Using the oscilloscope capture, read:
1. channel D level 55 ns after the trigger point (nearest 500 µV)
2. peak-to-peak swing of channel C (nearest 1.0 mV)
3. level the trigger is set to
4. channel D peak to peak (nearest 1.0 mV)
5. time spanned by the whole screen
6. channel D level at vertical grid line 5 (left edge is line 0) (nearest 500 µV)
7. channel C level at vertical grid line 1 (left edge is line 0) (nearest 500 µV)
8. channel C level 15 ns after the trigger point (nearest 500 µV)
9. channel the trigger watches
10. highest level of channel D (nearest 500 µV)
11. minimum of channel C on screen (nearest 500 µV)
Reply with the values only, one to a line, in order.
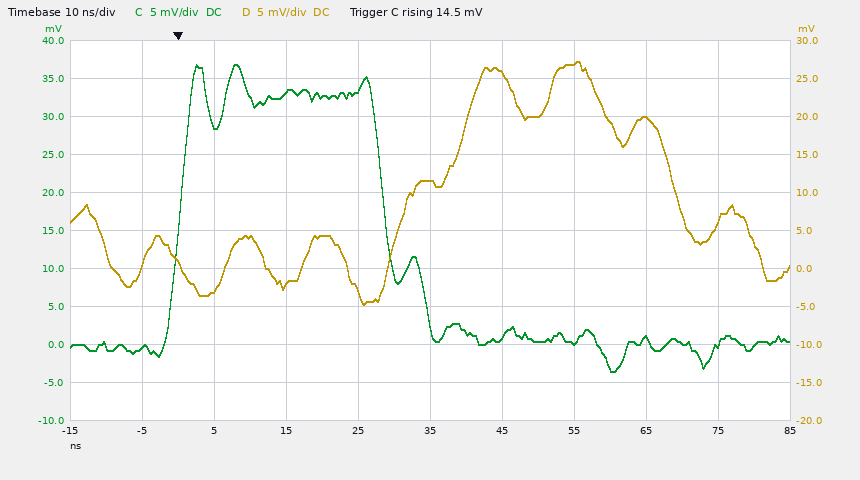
27.0 mV
40.0 mV
14.5 mV
32.0 mV
100 ns
11.5 mV
-500 µV
33.0 mV
channel C
27.0 mV
-3.5 mV
